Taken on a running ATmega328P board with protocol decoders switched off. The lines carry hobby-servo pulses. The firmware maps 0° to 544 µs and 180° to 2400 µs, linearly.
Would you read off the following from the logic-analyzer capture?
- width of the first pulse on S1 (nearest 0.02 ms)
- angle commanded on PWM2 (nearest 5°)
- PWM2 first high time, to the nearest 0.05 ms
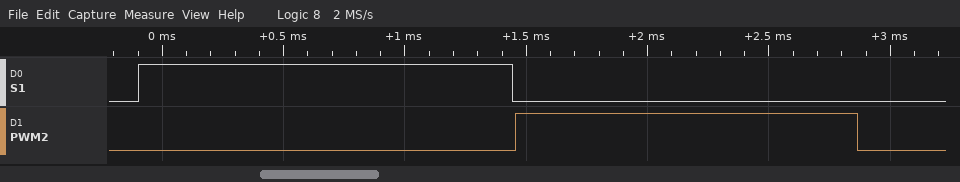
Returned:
1.54 ms
85°
1.40 ms
